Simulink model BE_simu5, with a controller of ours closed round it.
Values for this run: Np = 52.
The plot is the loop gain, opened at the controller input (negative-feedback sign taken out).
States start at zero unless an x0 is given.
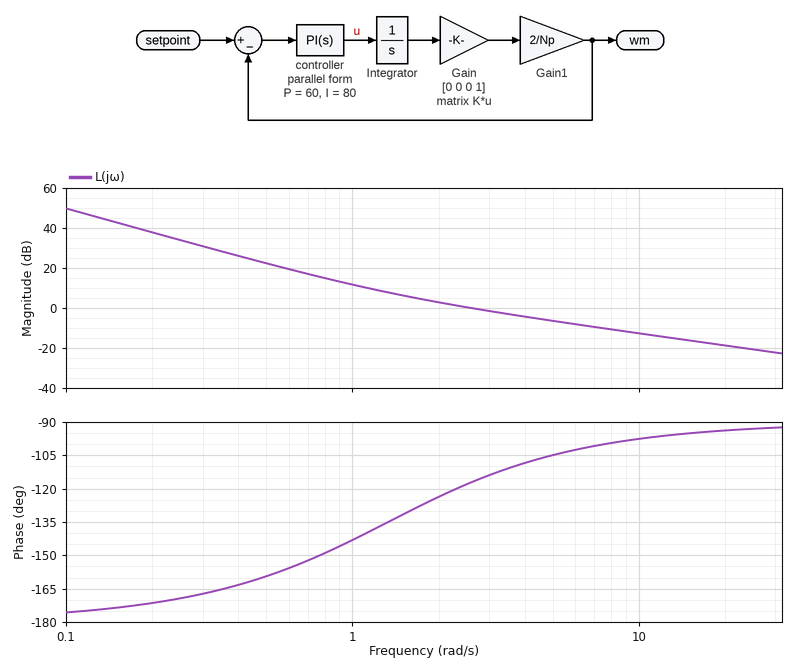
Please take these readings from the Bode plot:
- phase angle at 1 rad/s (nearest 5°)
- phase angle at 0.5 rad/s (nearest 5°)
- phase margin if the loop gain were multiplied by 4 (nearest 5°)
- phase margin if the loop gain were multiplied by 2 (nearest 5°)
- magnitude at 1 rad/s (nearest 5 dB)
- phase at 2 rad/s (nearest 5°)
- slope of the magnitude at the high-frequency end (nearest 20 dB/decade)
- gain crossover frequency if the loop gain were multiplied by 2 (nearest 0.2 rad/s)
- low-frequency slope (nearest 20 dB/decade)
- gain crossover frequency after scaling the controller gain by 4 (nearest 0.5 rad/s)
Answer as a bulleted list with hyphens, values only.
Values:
- -145°
- -160°
- 80°
- 75°
- 10 dB
- -125°
- -20 dB/decade
- 4.8 rad/s
- -40 dB/decade
- 9.5 rad/s
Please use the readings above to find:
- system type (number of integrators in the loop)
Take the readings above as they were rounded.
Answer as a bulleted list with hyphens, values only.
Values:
- 2
